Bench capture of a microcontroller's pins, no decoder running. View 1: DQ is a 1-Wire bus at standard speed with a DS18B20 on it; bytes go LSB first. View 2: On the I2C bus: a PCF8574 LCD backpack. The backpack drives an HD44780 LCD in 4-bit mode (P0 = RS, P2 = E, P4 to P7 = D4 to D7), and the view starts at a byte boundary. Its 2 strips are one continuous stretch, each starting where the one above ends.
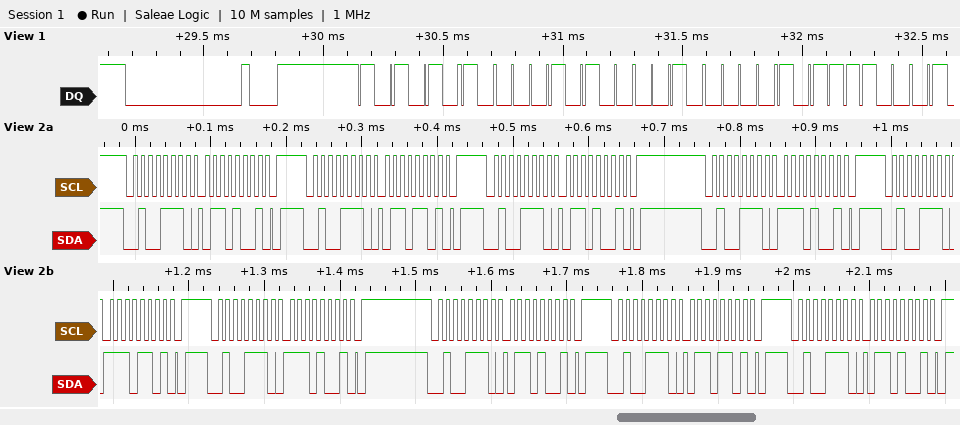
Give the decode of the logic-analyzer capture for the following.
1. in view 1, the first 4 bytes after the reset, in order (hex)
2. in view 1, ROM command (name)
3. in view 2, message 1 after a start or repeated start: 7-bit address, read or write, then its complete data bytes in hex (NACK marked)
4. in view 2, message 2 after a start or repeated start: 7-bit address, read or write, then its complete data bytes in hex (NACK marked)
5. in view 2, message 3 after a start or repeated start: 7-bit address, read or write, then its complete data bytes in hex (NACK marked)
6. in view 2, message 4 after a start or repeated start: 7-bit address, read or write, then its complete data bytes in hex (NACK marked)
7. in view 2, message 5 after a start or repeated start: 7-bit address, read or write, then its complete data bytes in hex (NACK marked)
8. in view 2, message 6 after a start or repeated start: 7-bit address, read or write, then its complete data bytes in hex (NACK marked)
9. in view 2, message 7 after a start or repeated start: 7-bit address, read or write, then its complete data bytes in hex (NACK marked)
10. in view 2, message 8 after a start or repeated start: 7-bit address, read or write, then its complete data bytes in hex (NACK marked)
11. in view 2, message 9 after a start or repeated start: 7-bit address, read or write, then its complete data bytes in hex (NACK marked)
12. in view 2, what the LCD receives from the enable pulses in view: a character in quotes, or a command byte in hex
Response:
55 28 04 3D
Match ROM
0x27 write: 69
0x27 write: 6D
0x27 write: 69
0x27 write: E9
0x27 write: ED
0x27 write: E9
0x27 write: 69
0x27 write: 6D
0x27 write: 69
'n'
